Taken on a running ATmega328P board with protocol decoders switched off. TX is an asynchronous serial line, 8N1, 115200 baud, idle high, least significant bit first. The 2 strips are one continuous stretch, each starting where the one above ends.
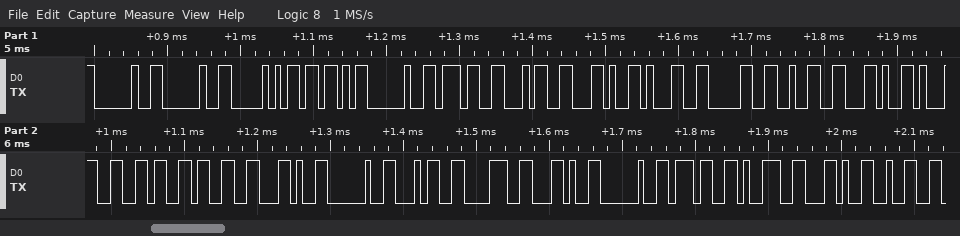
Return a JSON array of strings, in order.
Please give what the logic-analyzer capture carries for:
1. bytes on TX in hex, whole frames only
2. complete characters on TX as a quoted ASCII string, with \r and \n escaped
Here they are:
["20 20 50 5B 20 37 34 2C 31 30 32 2C 31 36 33 2C 20 34 38 2C 20 37 39 2C 32", "\"  P[ 74,102,163, 48, 79,2\""]
